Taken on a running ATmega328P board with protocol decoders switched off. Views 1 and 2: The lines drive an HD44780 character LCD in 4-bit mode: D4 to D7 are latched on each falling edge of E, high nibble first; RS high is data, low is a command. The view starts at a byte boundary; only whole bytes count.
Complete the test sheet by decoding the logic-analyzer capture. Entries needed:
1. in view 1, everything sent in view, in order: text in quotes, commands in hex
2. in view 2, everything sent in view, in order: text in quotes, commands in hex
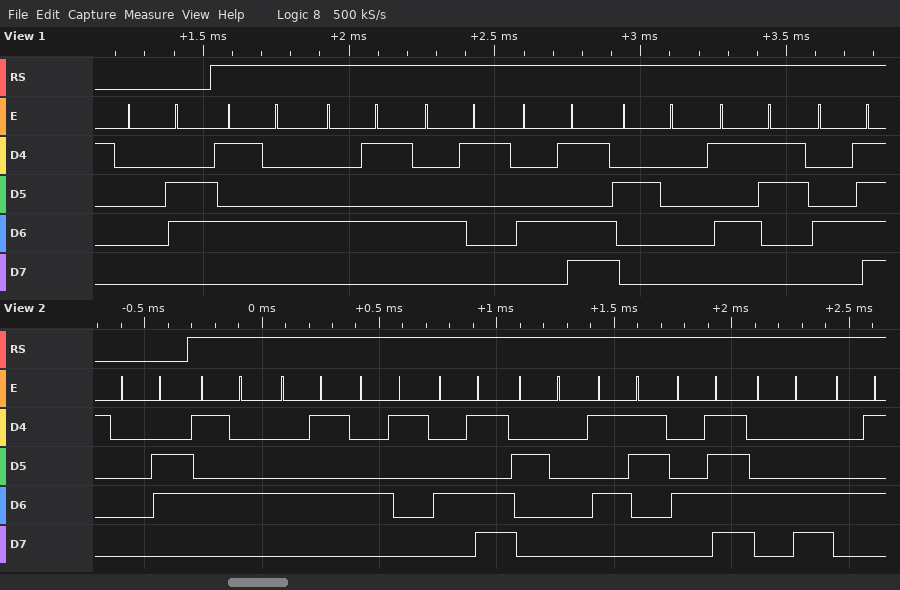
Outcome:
0x06 "TEAM SO"
0x06 "TEAM SOLE"
